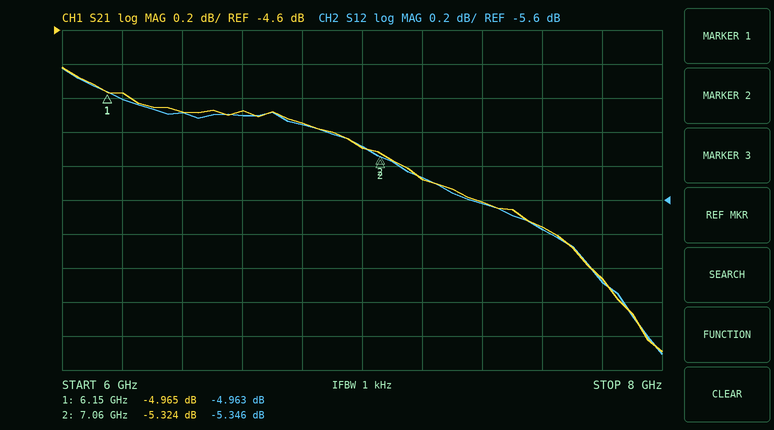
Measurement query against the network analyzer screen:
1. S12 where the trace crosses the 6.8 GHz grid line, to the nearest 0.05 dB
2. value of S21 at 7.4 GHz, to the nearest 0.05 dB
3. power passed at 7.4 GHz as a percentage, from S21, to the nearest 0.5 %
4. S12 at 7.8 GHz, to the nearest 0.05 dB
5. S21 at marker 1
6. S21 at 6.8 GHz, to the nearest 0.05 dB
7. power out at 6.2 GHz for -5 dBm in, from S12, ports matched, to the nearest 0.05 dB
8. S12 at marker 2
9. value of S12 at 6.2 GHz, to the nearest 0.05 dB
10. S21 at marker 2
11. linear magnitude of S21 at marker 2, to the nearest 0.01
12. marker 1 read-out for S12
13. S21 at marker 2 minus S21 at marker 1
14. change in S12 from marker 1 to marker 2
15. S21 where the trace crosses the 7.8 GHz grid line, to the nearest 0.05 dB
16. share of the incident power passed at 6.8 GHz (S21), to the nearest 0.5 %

-5.15 dB
-5.60 dB
27.5 %
-6.10 dB
-4.965 dB
-5.15 dB
-10.00 dBm
-5.346 dB
-5.00 dB
-5.324 dB
0.54
-4.963 dB
-0.359 dB
-0.383 dB
-6.05 dB
30.5 %
